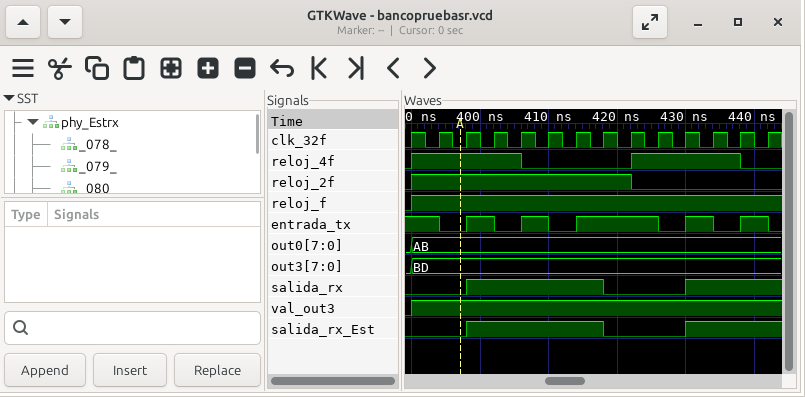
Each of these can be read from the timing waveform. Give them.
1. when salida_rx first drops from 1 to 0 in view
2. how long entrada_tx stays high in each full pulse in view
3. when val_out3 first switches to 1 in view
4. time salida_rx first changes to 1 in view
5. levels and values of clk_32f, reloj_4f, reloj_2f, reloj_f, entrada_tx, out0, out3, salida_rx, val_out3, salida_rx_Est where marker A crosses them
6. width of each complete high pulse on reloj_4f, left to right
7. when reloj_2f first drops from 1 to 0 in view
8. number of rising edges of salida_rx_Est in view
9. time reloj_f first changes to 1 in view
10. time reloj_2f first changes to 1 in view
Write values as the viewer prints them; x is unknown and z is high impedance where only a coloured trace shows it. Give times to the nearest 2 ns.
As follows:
418 ns
4 ns, 4 ns, 12 ns, 4 ns, 4 ns
390 ns
398 ns
clk_32f=0, reloj_4f=1, reloj_2f=1, reloj_f=1, entrada_tx=0, out0=AB, out3=BD, salida_rx=0, val_out3=1, salida_rx_Est=0
16 ns, 16 ns
422 ns
2
390 ns
390 ns
